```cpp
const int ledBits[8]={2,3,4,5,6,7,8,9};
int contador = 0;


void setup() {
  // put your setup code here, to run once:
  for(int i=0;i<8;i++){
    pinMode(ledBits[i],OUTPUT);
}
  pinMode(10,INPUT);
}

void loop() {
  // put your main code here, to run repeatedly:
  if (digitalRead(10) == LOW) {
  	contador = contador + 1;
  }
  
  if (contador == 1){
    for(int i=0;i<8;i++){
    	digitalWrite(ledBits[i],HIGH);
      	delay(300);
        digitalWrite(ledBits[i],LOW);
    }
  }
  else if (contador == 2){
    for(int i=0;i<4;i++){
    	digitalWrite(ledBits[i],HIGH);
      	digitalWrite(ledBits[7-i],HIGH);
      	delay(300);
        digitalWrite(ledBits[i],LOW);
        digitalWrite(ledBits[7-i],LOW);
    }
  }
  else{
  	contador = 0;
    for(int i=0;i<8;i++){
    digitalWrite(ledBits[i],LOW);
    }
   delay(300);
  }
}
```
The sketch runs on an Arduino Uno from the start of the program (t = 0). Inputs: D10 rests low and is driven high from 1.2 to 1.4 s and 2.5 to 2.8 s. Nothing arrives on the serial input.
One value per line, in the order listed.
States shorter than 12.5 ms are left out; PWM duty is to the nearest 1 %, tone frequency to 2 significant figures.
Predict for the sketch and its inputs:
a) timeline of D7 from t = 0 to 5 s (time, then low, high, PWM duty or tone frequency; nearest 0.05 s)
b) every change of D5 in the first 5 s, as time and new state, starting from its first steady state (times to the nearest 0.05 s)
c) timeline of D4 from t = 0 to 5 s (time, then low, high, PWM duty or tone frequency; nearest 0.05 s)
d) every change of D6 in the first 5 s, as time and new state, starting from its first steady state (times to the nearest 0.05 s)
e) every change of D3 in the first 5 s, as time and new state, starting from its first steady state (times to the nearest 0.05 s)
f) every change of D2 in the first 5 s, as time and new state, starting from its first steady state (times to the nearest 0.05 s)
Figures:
0 s low; 1.5 s high; 1.8 s low; 3 s high; 3.3 s low
0 s low; 0.9 s high; 1.2 s low; 3.3 s high; 3.6 s low; 4.8 s high
0 s low; 0.6 s high; 0.9 s low; 3 s high; 3.3 s low; 4.5 s high; 4.8 s low
0 s low; 1.2 s high; 1.5 s low; 3.3 s high; 3.6 s low
0 s low; 0.3 s high; 0.6 s low; 2.7 s high; 3 s low; 4.2 s high; 4.5 s low
0 s high; 0.3 s low; 2.4 s high; 2.7 s low; 3.9 s high; 4.2 s low
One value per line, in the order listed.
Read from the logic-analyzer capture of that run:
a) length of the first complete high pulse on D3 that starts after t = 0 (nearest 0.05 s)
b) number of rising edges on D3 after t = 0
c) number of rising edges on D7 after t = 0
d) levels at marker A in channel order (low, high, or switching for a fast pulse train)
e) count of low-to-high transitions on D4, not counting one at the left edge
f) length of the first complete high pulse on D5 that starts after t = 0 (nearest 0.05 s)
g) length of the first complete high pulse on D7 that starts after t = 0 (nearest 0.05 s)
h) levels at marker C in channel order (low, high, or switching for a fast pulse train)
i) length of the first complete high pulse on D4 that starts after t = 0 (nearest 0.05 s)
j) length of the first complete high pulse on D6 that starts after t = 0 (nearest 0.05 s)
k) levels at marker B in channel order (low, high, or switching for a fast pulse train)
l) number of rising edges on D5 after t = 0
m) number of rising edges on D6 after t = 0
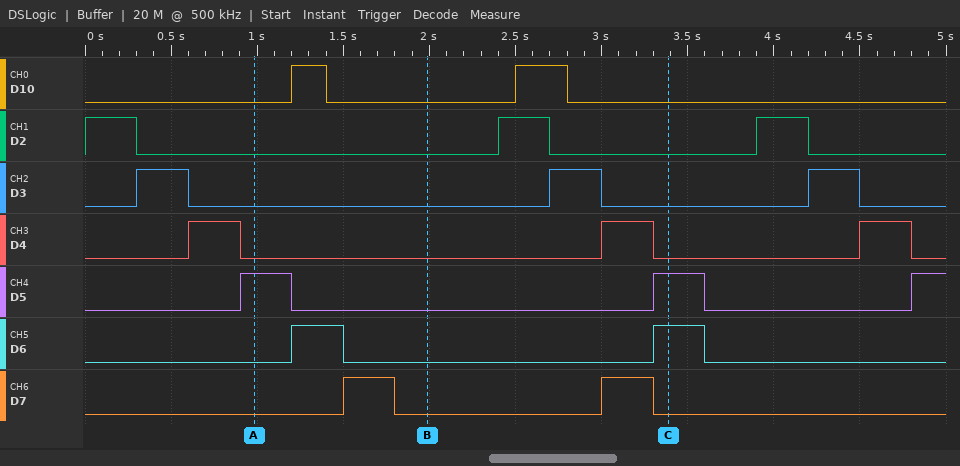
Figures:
0.30 s
3
2
D10 low, D2 low, D3 low, D4 low, D5 high, D6 low, D7 low
3
0.30 s
0.30 s
D10 low, D2 low, D3 low, D4 low, D5 high, D6 high, D7 low
0.30 s
0.30 s
D10 low, D2 low, D3 low, D4 low, D5 low, D6 low, D7 low
3
2
